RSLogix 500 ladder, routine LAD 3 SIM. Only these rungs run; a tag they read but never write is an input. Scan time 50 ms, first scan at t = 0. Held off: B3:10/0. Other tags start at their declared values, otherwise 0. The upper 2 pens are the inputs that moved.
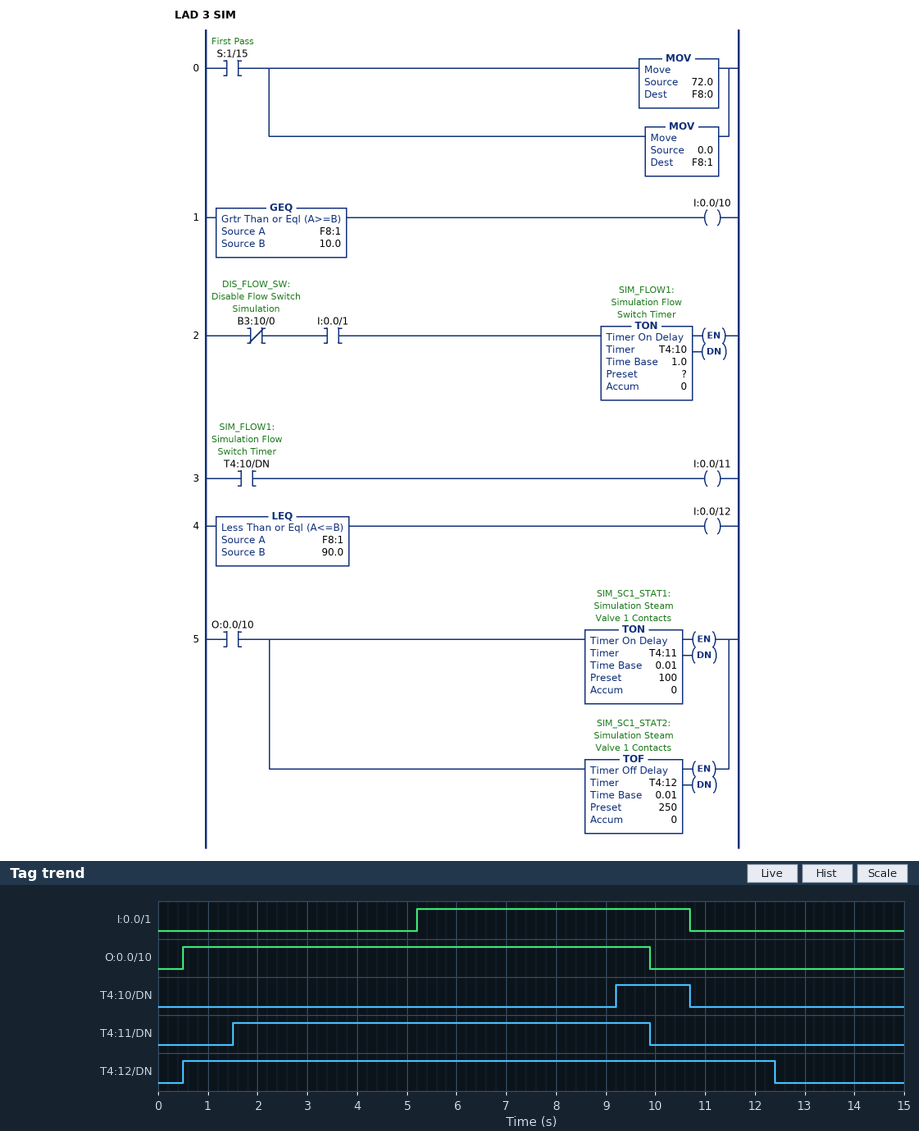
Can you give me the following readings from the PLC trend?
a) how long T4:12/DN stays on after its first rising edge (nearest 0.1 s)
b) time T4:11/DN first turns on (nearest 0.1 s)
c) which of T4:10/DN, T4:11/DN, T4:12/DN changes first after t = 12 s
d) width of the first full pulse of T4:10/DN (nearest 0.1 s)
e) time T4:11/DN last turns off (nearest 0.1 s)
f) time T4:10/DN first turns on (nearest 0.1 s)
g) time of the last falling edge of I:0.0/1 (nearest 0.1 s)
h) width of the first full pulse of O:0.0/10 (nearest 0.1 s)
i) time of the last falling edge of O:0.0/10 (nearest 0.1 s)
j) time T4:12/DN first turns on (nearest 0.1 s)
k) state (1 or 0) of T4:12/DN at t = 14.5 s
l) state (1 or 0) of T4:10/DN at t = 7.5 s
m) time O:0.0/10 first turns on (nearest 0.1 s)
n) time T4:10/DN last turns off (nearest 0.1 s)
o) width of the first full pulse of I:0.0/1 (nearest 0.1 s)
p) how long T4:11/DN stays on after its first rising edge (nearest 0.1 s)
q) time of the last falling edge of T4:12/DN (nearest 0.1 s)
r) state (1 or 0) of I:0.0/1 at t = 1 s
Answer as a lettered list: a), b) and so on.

a) 11.9 s
b) 1.5 s
c) T4:12/DN
d) 1.5 s
e) 9.9 s
f) 9.2 s
g) 10.7 s
h) 9.4 s
i) 9.9 s
j) 0.5 s
k) 0
l) 0
m) 0.5 s
n) 10.7 s
o) 5.5 s
p) 8.4 s
q) 12.4 s
r) 0
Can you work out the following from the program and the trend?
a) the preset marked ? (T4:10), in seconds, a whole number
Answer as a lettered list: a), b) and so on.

a) 4 s
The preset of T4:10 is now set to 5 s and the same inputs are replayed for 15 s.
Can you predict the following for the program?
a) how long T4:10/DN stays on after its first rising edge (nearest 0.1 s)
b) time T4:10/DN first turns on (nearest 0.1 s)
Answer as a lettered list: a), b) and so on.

a) 0.5 s
b) 10.2 s
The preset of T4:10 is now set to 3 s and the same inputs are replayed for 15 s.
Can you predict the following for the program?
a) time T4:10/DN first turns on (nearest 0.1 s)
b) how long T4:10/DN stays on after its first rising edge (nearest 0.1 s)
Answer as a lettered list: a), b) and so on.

a) 8.2 s
b) 2.5 s
